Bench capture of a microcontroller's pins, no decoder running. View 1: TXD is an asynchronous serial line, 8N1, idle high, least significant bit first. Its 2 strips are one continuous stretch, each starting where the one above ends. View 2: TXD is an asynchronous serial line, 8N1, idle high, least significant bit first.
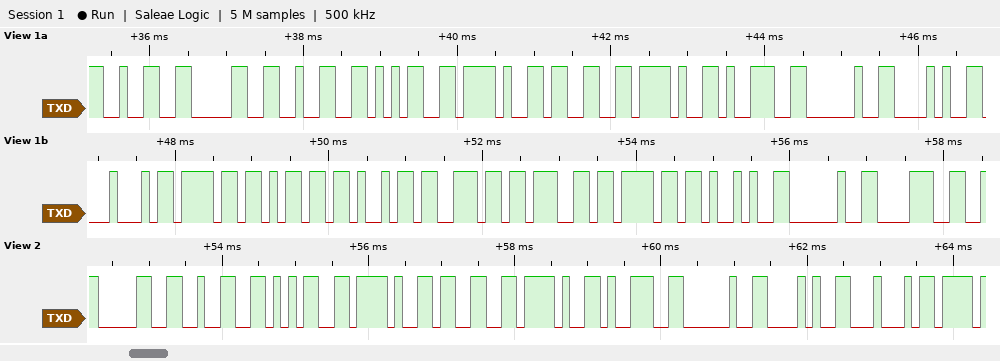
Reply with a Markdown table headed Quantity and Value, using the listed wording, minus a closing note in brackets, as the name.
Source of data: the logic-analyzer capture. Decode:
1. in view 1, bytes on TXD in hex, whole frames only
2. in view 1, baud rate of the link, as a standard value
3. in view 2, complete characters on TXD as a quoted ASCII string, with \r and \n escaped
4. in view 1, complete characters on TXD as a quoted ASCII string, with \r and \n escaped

| Quantity | Value |
|---|---|
| in view 1, bytes on TXD in hex, whole frames only | 32 30 32 35 2F 33 2F 39 20 28 44 6F 6D 69 6E 67 6F 29 20 38 |
| in view 1, baud rate of the link, as a standard value | 9600 baud |
| in view 2, complete characters on TXD as a quoted ASCII string, with \r and \n escaped | "025/3/9 (D" |
| in view 1, complete characters on TXD as a quoted ASCII string, with \r and \n escaped | "2025/3/9 (Domingo) 8" |
